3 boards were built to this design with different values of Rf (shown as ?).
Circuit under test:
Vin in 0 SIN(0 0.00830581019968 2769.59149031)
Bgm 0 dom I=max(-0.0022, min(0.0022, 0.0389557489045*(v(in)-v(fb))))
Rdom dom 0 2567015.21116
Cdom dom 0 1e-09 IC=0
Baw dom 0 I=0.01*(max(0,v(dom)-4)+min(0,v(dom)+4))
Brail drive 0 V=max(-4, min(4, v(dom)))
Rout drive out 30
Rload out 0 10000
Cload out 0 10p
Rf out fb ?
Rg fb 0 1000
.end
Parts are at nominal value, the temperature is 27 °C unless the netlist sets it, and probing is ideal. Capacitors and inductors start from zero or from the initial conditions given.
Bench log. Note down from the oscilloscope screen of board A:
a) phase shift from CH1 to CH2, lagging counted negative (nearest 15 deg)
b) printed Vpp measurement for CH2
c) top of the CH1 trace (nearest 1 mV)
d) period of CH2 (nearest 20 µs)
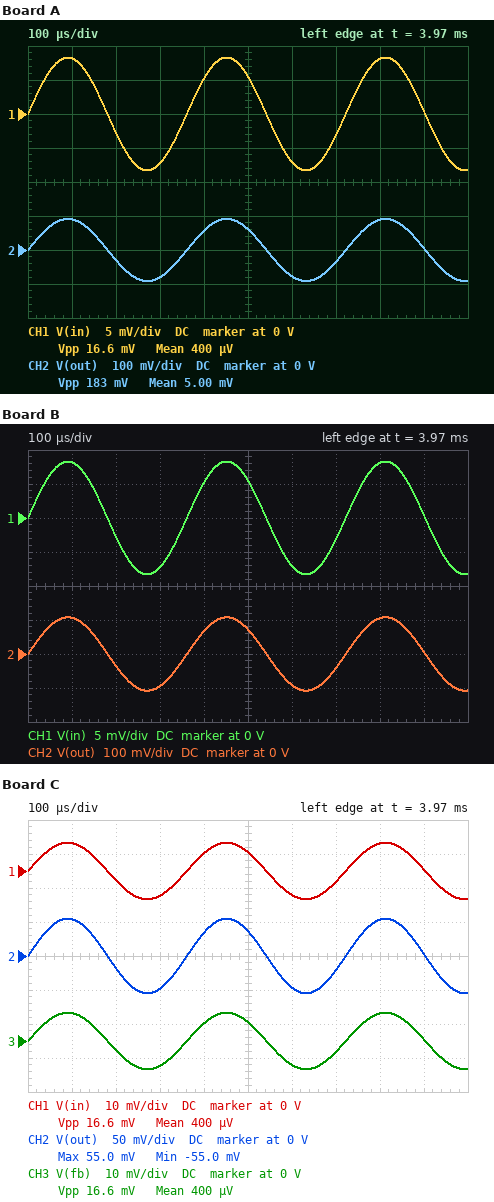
0 deg
183 mV
8 mV
360 µs
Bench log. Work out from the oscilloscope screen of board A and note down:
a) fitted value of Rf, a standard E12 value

10 kΩ
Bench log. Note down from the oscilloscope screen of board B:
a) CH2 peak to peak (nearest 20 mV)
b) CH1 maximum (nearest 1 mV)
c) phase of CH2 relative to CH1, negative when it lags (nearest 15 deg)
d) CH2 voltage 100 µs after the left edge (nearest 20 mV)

220 mV
8 mV
0 deg
100 mV
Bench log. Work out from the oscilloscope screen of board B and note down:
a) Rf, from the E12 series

12 kΩ
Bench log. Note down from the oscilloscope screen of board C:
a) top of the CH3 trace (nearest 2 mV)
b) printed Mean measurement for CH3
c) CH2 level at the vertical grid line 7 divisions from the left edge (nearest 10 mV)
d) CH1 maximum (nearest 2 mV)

8 mV
400 µV
-20 mV
8 mV
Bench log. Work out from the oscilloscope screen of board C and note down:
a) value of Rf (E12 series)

5.6 kΩ
